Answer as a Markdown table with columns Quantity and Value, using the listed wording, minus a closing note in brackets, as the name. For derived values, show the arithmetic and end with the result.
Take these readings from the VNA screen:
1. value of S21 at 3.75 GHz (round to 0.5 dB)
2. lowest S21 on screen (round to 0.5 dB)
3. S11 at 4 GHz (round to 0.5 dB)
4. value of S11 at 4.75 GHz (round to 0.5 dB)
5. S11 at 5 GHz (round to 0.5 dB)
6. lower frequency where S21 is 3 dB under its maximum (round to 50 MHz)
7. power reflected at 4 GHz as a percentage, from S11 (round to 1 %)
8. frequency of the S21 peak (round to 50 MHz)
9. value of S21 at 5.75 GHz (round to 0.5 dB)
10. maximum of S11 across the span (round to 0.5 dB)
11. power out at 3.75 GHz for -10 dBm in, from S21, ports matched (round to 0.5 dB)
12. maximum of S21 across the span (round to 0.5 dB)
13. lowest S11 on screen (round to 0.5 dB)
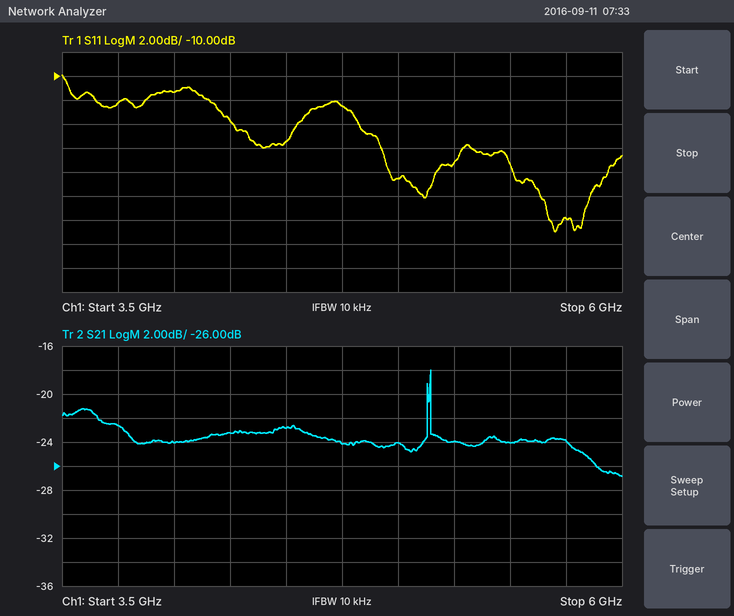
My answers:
| Quantity | Value |
|---|---|
| value of S21 at 3.75 GHz | -22.5 dB |
| lowest S21 on screen | -27.0 dB |
| S11 at 4 GHz | -11.5 dB |
| value of S11 at 4.75 GHz | -12.5 dB |
| S11 at 5 GHz | -18.5 dB |
| lower frequency where S21 is 3 dB under its maximum | 5.15 GHz |
| power reflected at 4 GHz as a percentage, from S11 | 10^(-11.5/10) ≈ 7 % |
| frequency of the S21 peak | 5.15 GHz |
| value of S21 at 5.75 GHz | -24.0 dB |
| maximum of S11 across the span | -10.0 dB |
| power out at 3.75 GHz for -10 dBm in, from S21, ports matched | -10 dBm + (-22.5 dB) = -32.5 dBm |
| maximum of S21 across the span | -18.0 dB |
| lowest S11 on screen | -23.0 dB |
